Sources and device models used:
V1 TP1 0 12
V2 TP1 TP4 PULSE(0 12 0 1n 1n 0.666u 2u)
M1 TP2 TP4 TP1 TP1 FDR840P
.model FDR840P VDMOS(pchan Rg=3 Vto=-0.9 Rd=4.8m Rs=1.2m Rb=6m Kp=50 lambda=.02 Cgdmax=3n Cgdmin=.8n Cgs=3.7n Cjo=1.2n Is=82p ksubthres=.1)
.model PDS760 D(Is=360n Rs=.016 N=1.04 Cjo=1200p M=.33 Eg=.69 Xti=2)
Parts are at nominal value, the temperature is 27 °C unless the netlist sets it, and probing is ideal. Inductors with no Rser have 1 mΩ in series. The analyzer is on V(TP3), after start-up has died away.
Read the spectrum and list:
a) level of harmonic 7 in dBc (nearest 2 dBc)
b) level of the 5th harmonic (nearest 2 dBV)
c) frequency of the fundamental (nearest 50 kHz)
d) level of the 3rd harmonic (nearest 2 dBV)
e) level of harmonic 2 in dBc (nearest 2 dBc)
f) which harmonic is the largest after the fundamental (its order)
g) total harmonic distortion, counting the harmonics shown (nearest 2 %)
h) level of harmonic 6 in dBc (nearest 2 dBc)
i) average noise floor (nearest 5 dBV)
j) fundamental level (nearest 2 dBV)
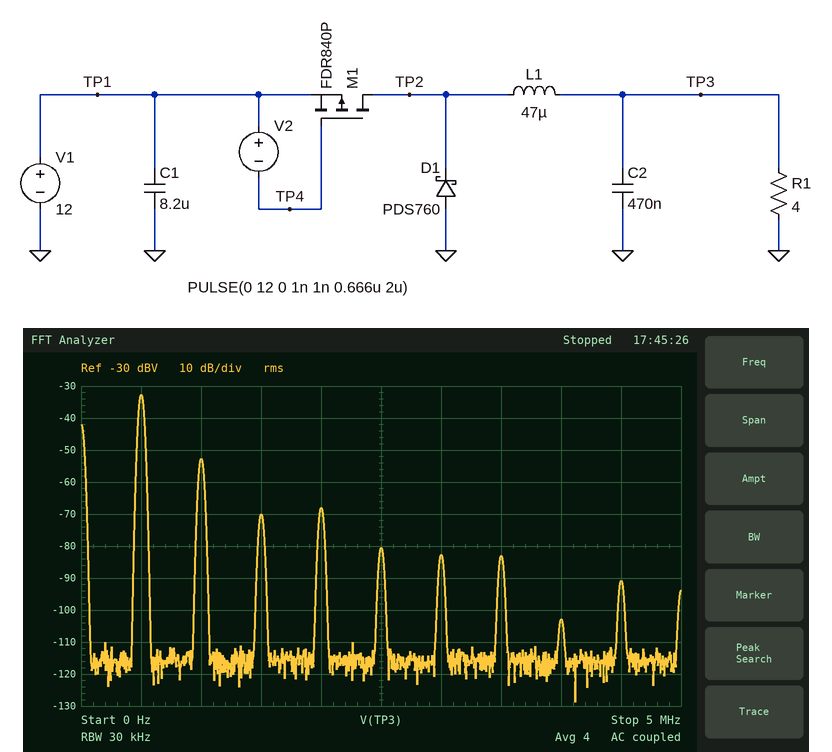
-50 dBc
-80 dBV
500 kHz
-70 dBV
-20 dBc
2
10 %
-50 dBc
-115 dBV
-32 dBV
